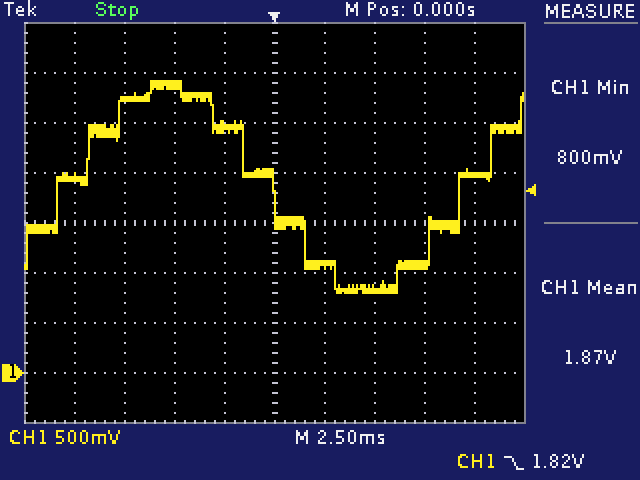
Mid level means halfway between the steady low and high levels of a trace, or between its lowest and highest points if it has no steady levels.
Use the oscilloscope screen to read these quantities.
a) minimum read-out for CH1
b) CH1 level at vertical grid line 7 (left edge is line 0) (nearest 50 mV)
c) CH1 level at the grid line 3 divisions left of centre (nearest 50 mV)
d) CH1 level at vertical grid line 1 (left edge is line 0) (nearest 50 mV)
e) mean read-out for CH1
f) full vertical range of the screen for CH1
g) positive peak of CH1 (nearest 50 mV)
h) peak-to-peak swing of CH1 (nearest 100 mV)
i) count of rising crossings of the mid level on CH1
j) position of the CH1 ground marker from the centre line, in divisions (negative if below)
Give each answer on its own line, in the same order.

800 mV
850 mV
2.75 V
1.95 V
1.87 V
4 V
2.90 V
2.10 V
2
-3.0 div
